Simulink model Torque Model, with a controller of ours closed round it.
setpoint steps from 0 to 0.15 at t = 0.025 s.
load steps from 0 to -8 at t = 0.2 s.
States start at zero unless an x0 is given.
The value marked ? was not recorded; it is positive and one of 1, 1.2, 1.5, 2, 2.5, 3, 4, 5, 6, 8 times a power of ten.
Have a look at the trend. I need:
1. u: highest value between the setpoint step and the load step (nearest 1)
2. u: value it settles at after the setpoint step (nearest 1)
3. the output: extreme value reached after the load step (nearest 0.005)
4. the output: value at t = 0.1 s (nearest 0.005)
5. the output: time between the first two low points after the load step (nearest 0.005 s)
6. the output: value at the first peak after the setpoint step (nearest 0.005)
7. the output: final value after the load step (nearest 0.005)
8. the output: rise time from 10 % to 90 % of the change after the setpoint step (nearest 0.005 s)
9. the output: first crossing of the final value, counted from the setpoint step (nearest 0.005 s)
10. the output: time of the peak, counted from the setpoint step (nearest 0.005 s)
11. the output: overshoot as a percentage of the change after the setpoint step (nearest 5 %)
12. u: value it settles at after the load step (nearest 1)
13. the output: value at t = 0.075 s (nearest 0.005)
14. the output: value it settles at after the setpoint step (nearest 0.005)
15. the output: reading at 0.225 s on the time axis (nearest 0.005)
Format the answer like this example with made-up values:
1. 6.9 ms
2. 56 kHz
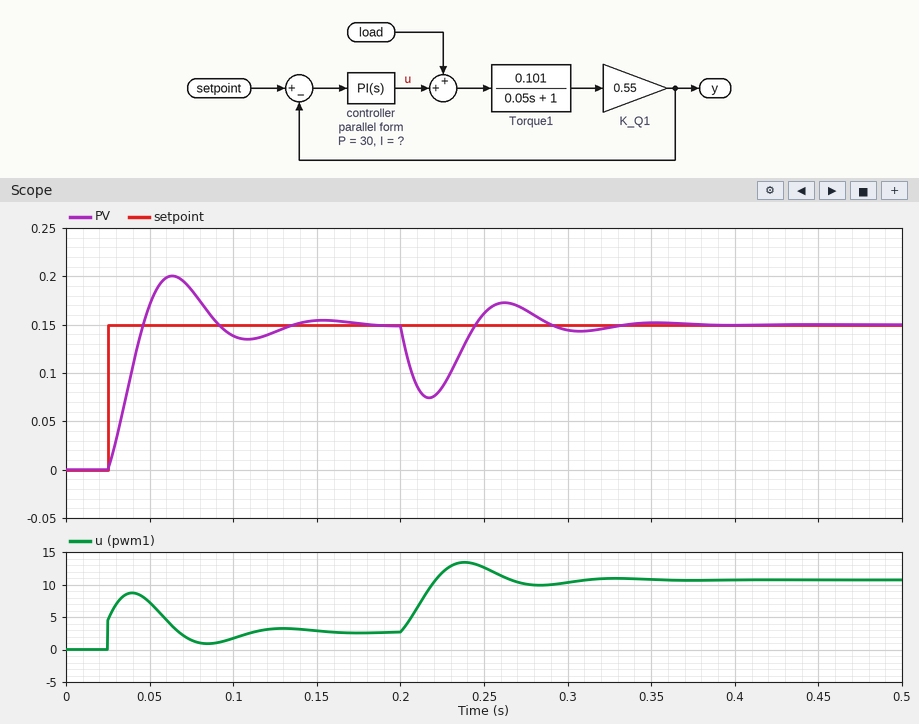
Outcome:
1. 9
2. 3
3. 0.075
4. 0.140
5. 0.090 s
6. 0.200
7. 0.150
8. 0.015 s
9. 0.020 s
10. 0.040 s
11. 35 %
12. 11
13. 0.185
14. 0.150
15. 0.085
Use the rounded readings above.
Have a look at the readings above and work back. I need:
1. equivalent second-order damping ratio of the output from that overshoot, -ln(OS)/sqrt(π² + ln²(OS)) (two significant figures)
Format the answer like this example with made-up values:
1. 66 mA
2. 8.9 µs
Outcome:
1. 0.32
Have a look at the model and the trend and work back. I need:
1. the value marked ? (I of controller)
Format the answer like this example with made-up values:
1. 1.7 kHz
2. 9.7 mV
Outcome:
1. 5000
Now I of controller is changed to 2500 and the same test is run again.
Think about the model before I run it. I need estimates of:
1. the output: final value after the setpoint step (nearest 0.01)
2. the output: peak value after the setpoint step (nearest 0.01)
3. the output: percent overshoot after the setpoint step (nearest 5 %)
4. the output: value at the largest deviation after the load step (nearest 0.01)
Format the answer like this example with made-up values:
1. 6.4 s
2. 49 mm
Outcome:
1. 0.15
2. 0.18
3. 20 %
4. 0.06
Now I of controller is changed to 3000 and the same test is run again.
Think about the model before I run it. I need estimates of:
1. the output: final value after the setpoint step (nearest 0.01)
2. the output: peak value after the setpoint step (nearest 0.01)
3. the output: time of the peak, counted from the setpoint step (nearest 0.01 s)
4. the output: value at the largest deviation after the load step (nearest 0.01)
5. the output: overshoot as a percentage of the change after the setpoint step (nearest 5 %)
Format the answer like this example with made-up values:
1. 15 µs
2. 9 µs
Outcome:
1. 0.15
2. 0.19
3. 0.05 s
4. 0.06
5. 25 %
